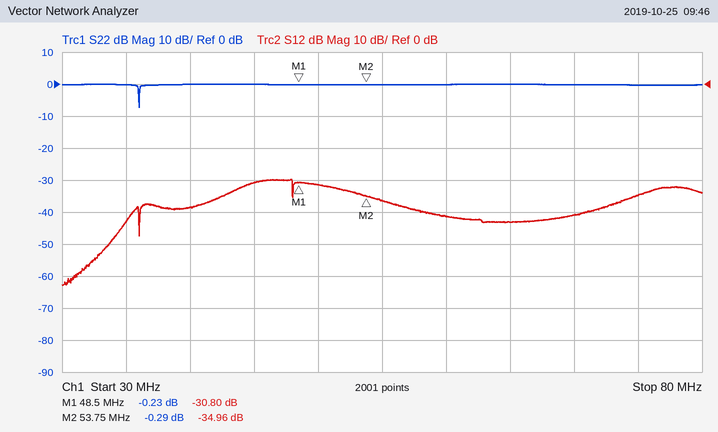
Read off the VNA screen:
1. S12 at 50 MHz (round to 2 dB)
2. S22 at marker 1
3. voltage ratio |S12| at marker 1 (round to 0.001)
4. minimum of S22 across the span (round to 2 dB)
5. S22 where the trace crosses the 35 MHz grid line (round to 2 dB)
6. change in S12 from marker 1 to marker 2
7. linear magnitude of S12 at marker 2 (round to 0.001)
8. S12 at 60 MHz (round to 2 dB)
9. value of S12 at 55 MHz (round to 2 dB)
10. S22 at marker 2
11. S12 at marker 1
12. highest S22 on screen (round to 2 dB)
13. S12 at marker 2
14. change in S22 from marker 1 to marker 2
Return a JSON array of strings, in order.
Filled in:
["-32 dB", "-0.23 dB", "0.029", "-8 dB", "0 dB", "-4.16 dB", "0.018", "-42 dB", "-36 dB", "-0.29 dB", "-30.80 dB", "0 dB", "-34.96 dB", "-0.06 dB"]
